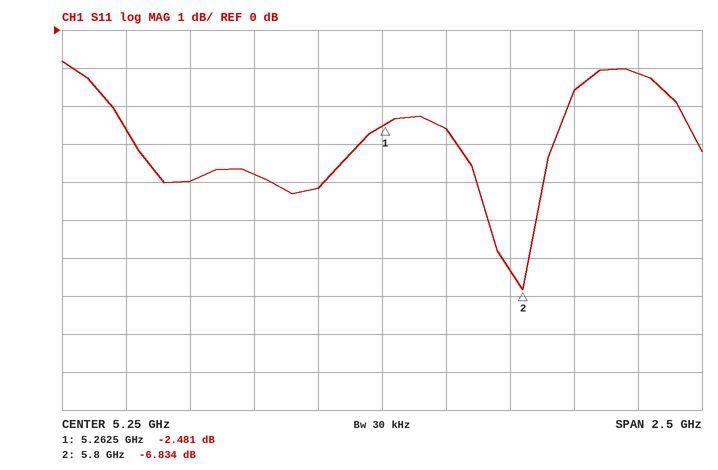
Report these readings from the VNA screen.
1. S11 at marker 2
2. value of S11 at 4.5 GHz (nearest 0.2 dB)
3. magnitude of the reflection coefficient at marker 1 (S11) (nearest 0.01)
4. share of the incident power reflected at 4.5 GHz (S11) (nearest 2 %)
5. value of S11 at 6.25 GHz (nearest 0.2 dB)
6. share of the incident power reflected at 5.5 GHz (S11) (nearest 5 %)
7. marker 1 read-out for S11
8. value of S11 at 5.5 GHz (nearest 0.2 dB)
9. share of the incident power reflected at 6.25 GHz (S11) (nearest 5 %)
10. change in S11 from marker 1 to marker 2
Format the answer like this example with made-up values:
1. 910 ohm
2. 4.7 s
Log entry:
1. -6.834 dB
2. -4.0 dB
3. 0.75
4. 40 %
5. -1.2 dB
6. 55 %
7. -2.481 dB
8. -2.6 dB
9. 75 %
10. -4.353 dB
